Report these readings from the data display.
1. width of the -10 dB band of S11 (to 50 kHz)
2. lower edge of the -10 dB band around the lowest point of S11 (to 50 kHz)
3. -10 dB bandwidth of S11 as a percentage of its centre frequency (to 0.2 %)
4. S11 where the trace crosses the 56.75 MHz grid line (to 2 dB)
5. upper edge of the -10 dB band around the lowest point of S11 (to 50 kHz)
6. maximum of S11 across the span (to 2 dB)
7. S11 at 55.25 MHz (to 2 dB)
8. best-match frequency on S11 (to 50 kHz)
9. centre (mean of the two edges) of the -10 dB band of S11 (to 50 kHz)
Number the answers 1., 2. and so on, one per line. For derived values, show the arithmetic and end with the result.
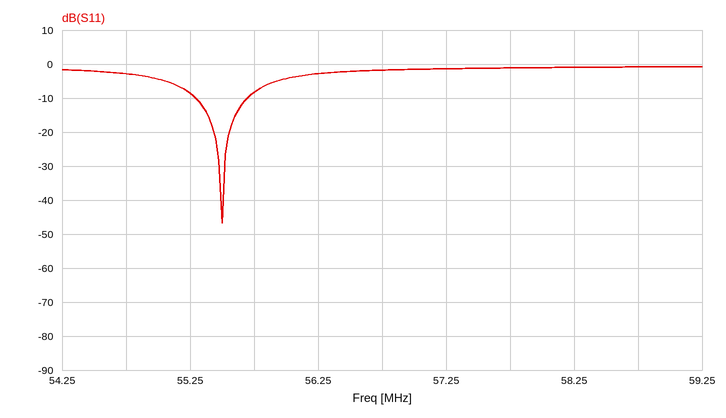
1. 55.70 MHz − 55.30 MHz = 400 kHz
2. 55.30 MHz
3. 400 kHz / 55.5 MHz ≈ 0.721 %, so 0.8 % to the nearest 0.2 %
4. -2 dB
5. 55.70 MHz
6. 0 dB
7. -8 dB
8. 55.50 MHz
9. 55.50 MHz
